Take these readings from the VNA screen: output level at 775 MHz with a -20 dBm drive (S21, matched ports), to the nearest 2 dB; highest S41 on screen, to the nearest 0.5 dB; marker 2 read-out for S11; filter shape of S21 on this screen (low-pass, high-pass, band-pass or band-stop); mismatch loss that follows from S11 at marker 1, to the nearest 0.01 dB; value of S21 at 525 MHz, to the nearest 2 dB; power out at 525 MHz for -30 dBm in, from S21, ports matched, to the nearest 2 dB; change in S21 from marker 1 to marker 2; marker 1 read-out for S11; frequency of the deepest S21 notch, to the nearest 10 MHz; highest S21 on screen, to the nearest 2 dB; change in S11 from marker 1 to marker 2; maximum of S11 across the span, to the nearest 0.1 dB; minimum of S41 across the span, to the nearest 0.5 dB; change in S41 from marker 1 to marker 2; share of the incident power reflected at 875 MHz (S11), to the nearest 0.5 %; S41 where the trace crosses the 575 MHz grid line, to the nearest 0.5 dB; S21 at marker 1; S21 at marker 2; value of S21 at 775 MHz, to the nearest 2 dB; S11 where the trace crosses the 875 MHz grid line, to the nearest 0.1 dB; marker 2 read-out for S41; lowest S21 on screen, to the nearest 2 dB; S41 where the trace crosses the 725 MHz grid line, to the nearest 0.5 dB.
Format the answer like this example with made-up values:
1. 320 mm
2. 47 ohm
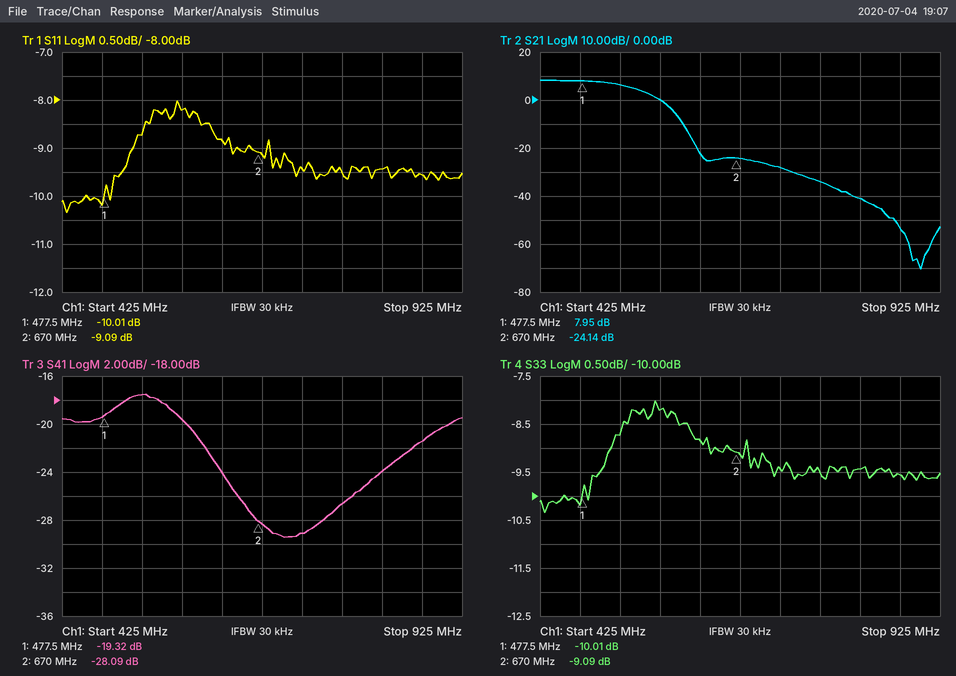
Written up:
1. -54 dBm
2. -17.5 dB
3. -9.09 dB
4. low-pass
5. 0.46 dB
6. 6 dB
7. -24 dBm
8. -32.09 dB
9. -10.01 dB
10. 900 MHz
11. 8 dB
12. 0.92 dB
13. -8.0 dB
14. -29.5 dB
15. -8.77 dB
16. 11.0 %
17. -19.5 dB
18. 7.95 dB
19. -24.14 dB
20. -34 dB
21. -9.6 dB
22. -28.09 dB
23. -70 dB
24. -29.0 dB
